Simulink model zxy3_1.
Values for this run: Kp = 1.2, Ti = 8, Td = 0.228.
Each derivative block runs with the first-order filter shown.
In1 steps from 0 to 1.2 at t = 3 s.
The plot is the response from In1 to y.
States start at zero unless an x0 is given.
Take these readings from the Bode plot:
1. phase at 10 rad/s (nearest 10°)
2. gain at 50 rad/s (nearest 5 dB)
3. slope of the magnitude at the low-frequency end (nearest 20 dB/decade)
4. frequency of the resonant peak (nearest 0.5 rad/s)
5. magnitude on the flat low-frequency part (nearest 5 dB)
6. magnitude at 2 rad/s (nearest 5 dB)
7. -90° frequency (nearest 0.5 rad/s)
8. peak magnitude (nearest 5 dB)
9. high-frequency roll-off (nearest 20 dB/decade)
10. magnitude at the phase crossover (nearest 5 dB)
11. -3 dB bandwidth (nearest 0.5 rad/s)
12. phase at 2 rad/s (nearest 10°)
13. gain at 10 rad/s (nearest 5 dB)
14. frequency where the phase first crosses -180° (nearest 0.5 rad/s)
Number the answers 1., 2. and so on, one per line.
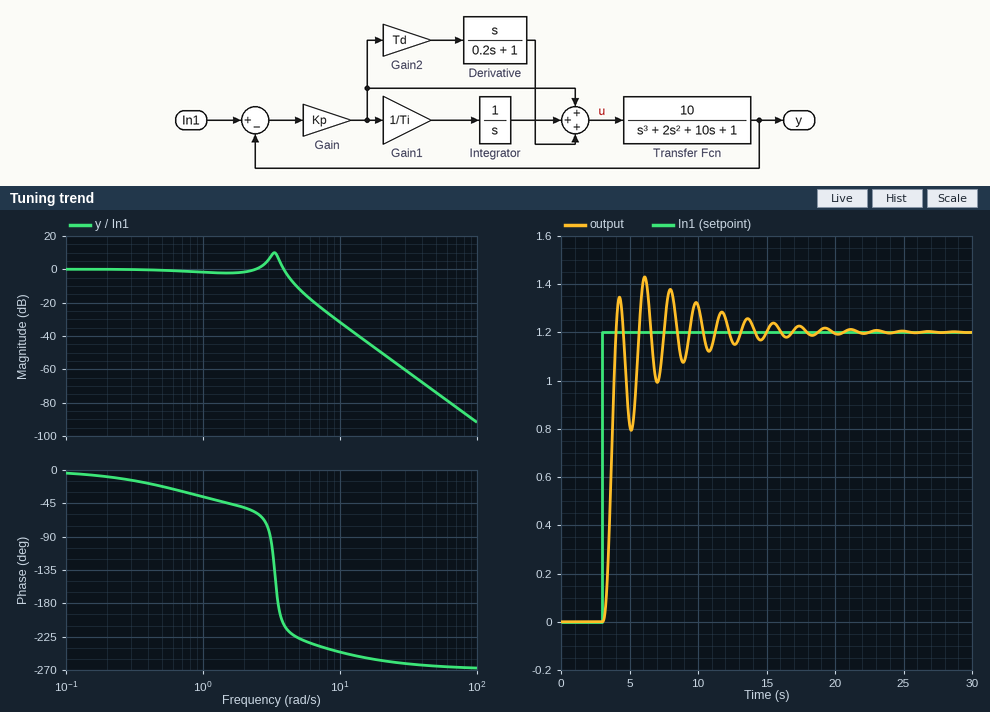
1. -250°
2. -75 dB
3. 0 dB/decade
4. 3.5 rad/s
5. 0 dB
6. 0 dB
7. 3.0 rad/s
8. 10 dB
9. -60 dB/decade
10. 5 dB
11. 4.0 rad/s
12. -50°
13. -30 dB
14. 3.5 rad/s
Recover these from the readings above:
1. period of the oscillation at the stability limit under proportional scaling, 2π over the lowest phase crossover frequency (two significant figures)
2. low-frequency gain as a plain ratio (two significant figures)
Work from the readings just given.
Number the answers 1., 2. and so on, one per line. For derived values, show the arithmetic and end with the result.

1. 2π / 3.5 = 1.8 s
2. 10^(0 / 20) = 1.0
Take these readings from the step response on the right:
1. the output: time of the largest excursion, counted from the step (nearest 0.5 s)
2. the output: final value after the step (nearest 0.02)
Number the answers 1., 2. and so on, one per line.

1. 3.0 s
2. 1.20
